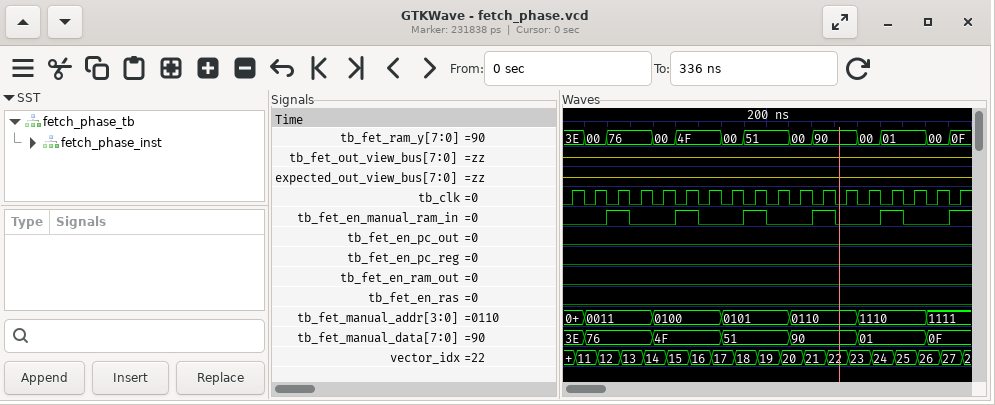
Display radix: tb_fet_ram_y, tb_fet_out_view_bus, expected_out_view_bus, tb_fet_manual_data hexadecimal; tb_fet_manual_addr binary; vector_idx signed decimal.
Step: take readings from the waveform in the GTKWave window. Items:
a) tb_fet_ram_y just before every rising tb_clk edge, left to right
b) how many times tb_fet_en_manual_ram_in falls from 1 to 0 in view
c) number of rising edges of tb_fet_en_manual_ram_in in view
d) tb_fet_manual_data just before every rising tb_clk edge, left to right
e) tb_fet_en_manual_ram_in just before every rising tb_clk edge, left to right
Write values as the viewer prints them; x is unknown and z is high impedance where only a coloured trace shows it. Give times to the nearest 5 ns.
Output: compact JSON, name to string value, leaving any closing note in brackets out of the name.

{"tb_fet_ram_y just before every rising tb_clk edge, left to right": "3E, 00, 76, 76, 00, 4F, 4F, 00, 51, 51, 00, 90, 90, 00, 01, 01, 00, 0F", "how many times tb_fet_en_manual_ram_in falls from 1 to 0 in view": "5", "number of rising edges of tb_fet_en_manual_ram_in in view": "6", "tb_fet_manual_data just before every rising tb_clk edge, left to right": "3E, 76, 76, 76, 4F, 4F, 4F, 51, 51, 51, 90, 90, 90, 01, 01, 01, 0F, 0F", "tb_fet_en_manual_ram_in just before every rising tb_clk edge, left to right": "0 0 1 0 0 1 0 0 1 0 0 1 0 0 1 0 0 1"}
